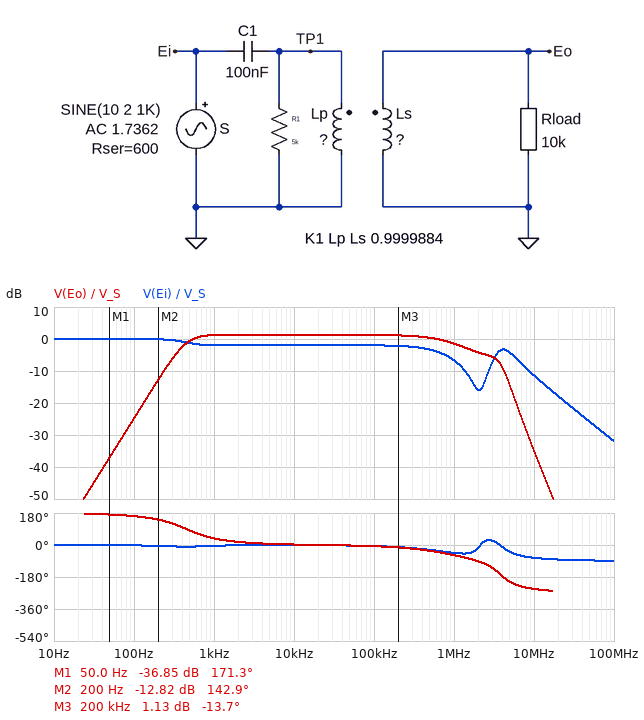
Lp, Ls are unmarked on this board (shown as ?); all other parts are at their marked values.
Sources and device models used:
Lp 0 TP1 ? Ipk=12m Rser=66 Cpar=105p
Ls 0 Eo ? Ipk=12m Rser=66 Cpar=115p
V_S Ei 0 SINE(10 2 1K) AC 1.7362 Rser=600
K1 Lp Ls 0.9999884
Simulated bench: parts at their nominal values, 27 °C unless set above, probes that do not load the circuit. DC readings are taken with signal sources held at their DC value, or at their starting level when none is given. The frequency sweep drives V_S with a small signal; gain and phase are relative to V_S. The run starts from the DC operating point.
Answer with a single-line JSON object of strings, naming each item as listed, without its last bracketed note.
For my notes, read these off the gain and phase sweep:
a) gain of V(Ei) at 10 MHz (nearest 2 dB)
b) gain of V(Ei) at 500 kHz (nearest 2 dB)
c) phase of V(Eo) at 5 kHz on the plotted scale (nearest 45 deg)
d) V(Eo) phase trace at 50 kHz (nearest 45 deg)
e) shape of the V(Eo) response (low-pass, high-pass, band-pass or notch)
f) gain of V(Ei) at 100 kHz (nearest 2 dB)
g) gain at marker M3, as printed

{"gain of V(Ei) at 10 MHz": "-12 dB", "gain of V(Ei) at 500 kHz": "-4 dB", "phase of V(Eo) at 5 kHz on the plotted scale": "0 deg", "V(Eo) phase trace at 50 kHz": "0 deg", "shape of the V(Eo) response": "band-pass", "gain of V(Ei) at 100 kHz": "-2 dB", "gain at marker M3, as printed": "1.13 dB"}
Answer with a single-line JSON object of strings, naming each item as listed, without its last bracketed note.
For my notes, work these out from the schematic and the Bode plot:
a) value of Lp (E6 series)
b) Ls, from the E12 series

{"value of Lp": "1 H", "Ls, from the E12 series": "2.2 H"}
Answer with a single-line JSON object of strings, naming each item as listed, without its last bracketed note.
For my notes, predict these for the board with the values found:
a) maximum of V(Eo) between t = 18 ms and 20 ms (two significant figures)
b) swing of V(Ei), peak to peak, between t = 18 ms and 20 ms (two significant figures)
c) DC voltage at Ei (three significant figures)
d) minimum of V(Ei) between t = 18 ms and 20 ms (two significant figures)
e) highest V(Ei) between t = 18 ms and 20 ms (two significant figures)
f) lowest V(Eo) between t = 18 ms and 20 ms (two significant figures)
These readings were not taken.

{"maximum of V(Eo) between t = 18 ms and 20 ms": "2.3 V", "swing of V(Ei), peak to peak, between t = 18 ms and 20 ms": "3.2 V", "DC voltage at Ei": "10.0 V", "minimum of V(Ei) between t = 18 ms and 20 ms": "8.4 V", "highest V(Ei) between t = 18 ms and 20 ms": "12 V", "lowest V(Eo) between t = 18 ms and 20 ms": "-2.3 V"}
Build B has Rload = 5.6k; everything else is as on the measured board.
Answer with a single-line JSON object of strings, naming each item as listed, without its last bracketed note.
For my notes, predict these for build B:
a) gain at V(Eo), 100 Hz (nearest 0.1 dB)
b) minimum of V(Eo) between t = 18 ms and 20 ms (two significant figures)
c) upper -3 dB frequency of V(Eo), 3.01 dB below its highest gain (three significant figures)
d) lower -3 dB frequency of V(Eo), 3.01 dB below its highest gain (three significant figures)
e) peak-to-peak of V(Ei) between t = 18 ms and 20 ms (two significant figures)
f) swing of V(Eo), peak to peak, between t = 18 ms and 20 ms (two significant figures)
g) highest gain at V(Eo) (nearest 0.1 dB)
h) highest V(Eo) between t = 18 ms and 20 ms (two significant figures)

{"gain at V(Eo), 100 Hz": "-25.1 dB", "minimum of V(Eo) between t = 18 ms and 20 ms": "-1.9 V", "upper -3 dB frequency of V(Eo), 3.01 dB below its highest gain": "1.20 MHz", "lower -3 dB frequency of V(Eo), 3.01 dB below its highest gain": "561 Hz", "peak-to-peak of V(Ei) between t = 18 ms and 20 ms": "3.2 V", "swing of V(Eo), peak to peak, between t = 18 ms and 20 ms": "3.8 V", "highest gain at V(Eo)": "0.5 dB", "highest V(Eo) between t = 18 ms and 20 ms": "1.9 V"}
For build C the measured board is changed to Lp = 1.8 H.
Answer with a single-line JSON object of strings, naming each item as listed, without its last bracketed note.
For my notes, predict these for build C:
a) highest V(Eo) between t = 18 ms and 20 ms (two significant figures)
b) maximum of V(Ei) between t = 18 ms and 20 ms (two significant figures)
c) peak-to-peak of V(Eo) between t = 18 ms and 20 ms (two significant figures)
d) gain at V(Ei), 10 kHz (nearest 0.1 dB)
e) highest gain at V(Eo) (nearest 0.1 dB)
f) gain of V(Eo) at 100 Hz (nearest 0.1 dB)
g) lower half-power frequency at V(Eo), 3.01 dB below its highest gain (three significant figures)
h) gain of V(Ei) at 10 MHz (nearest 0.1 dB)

{"highest V(Eo) between t = 18 ms and 20 ms": "1.8 V", "maximum of V(Ei) between t = 18 ms and 20 ms": "12 V", "peak-to-peak of V(Eo) between t = 18 ms and 20 ms": "3.6 V", "gain at V(Ei), 10 kHz": "-1.5 dB", "highest gain at V(Eo)": "-0.8 dB", "gain of V(Eo) at 100 Hz": "-22.3 dB", "lower half-power frequency at V(Eo), 3.01 dB below its highest gain": "337 Hz", "gain of V(Ei) at 10 MHz": "-11.8 dB"}
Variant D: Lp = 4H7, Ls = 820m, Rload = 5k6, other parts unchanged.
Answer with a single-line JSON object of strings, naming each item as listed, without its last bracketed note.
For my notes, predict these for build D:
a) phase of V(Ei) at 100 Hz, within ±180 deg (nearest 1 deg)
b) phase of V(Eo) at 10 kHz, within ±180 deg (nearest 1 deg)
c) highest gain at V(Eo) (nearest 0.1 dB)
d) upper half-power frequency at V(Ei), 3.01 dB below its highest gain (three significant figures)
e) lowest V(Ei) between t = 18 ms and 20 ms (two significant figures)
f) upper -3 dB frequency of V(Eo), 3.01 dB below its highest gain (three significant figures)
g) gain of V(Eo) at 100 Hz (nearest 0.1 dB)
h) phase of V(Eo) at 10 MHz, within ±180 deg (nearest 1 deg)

{"phase of V(Ei) at 100 Hz, within ±180 deg": "-2 deg", "phase of V(Eo) at 10 kHz, within ±180 deg": "2 deg", "highest gain at V(Eo)": "-3.8 dB", "upper half-power frequency at V(Ei), 3.01 dB below its highest gain": "1.64 MHz", "lowest V(Ei) between t = 18 ms and 20 ms": "8.2 V", "upper -3 dB frequency of V(Eo), 3.01 dB below its highest gain": "4.03 MHz", "gain of V(Eo) at 100 Hz": "-23.0 dB", "phase of V(Eo) at 10 MHz, within ±180 deg": "112 deg"}
